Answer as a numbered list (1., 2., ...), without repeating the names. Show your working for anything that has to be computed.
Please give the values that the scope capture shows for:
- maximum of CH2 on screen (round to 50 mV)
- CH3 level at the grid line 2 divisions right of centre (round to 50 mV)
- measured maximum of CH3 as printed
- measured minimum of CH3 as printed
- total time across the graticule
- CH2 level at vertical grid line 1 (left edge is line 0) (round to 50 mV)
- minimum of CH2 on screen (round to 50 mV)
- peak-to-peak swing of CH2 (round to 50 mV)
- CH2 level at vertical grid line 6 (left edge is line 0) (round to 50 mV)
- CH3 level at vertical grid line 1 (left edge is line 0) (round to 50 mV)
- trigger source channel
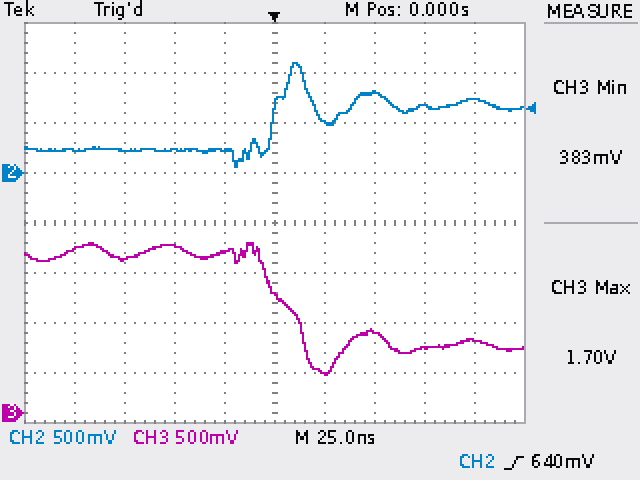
1. 1.10 V
2. 800 mV
3. 1.70 V
4. 383 mV
5. 250 ns
6. 250 mV
7. 50 mV
8. 1.10 V − (50 mV) = 1.05 V
9. 500 mV
10. 1.65 V
11. CH2
